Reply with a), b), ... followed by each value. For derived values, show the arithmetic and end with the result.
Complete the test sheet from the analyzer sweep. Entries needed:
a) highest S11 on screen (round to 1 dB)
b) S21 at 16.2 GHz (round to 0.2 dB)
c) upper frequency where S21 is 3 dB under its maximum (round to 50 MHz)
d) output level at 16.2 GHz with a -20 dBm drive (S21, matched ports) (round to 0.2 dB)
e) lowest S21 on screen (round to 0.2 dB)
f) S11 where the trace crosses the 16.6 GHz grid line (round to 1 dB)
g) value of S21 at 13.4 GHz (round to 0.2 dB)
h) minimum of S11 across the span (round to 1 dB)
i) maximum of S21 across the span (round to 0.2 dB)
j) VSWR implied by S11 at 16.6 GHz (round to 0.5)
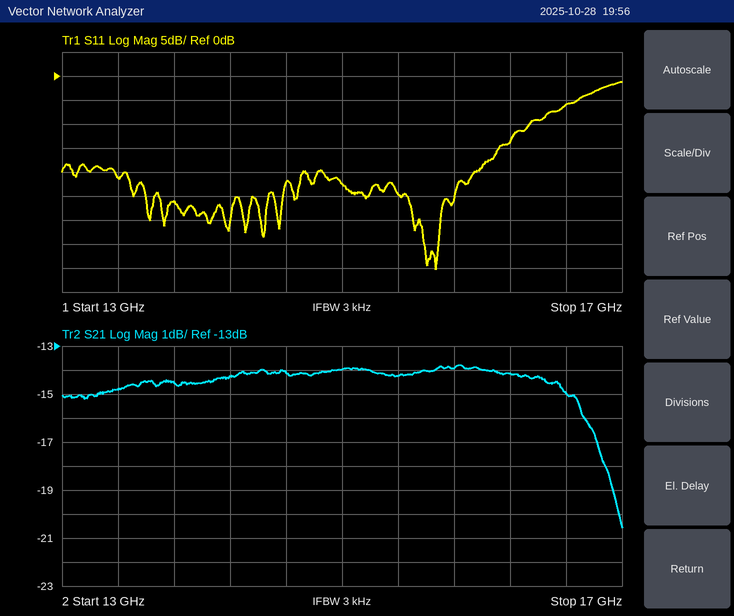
a) -1 dB
b) -14.2 dB
c) 16.80 GHz
d) -20 dBm + (-14.2 dB) = -34.2 dBm
e) -20.6 dB
f) -6 dB
g) -14.8 dB
h) -40 dB
i) -13.8 dB
j) |Γ| = 10^(-6/20) = 0.5012; VSWR = (1 + 0.5012)/(1 − 0.5012) ≈ 3.0
